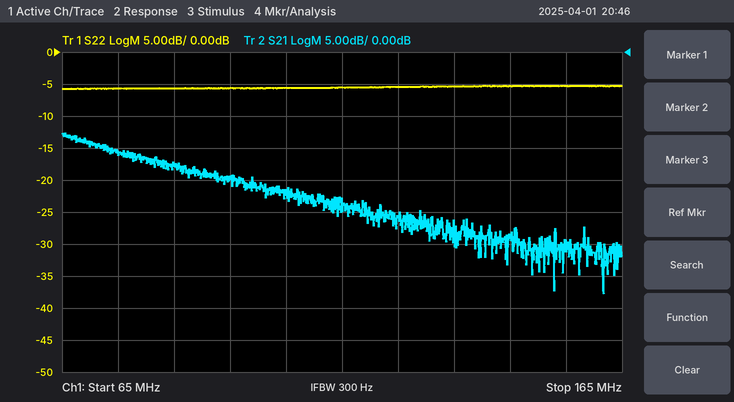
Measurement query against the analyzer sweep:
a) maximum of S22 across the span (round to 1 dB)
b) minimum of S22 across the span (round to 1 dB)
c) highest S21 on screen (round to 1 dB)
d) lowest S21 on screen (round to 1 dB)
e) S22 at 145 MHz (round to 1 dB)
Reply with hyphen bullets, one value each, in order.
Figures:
- -5 dB
- -6 dB
- -13 dB
- -38 dB
- -5 dB
